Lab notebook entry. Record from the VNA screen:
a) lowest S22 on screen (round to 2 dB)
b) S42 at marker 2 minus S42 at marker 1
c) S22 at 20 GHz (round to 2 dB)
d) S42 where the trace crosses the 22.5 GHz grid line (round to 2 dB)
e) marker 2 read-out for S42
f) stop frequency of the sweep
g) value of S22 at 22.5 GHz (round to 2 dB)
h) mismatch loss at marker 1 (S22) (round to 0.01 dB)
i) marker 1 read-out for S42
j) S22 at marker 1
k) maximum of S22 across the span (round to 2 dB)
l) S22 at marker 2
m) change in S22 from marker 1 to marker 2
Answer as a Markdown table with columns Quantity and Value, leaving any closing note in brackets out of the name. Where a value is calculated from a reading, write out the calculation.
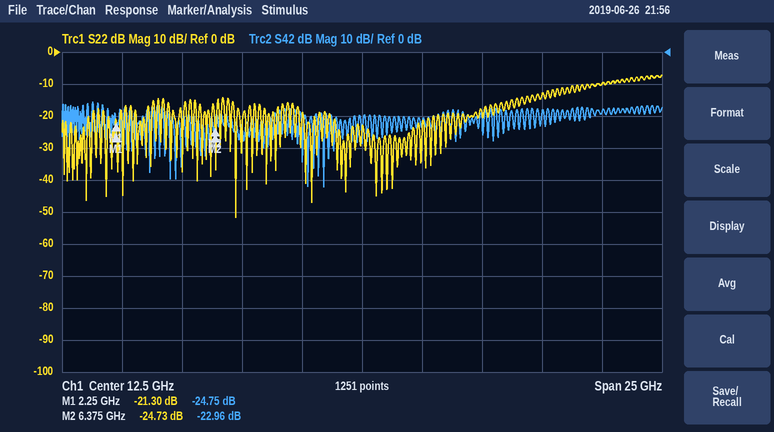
| Quantity | Value |
|---|---|
| lowest S22 on screen | -52 dB |
| S42 at marker 2 minus S42 at marker 1 | -22.96 − (-24.75) = 1.79 dB |
| S22 at 20 GHz | -14 dB |
| S42 where the trace crosses the 22.5 GHz grid line | -18 dB |
| marker 2 read-out for S42 | -22.96 dB |
| stop frequency of the sweep | 25 GHz |
| value of S22 at 22.5 GHz | -10 dB |
| mismatch loss at marker 1 (S22) | −10 log10(1 − 10^(-21.3/10)) ≈ 0.03 dB |
| marker 1 read-out for S42 | -24.75 dB |
| S22 at marker 1 | -21.30 dB |
| maximum of S22 across the span | -8 dB |
| S22 at marker 2 | -24.73 dB |
| change in S22 from marker 1 to marker 2 | -24.73 − (-21.3) = -3.43 dB |
